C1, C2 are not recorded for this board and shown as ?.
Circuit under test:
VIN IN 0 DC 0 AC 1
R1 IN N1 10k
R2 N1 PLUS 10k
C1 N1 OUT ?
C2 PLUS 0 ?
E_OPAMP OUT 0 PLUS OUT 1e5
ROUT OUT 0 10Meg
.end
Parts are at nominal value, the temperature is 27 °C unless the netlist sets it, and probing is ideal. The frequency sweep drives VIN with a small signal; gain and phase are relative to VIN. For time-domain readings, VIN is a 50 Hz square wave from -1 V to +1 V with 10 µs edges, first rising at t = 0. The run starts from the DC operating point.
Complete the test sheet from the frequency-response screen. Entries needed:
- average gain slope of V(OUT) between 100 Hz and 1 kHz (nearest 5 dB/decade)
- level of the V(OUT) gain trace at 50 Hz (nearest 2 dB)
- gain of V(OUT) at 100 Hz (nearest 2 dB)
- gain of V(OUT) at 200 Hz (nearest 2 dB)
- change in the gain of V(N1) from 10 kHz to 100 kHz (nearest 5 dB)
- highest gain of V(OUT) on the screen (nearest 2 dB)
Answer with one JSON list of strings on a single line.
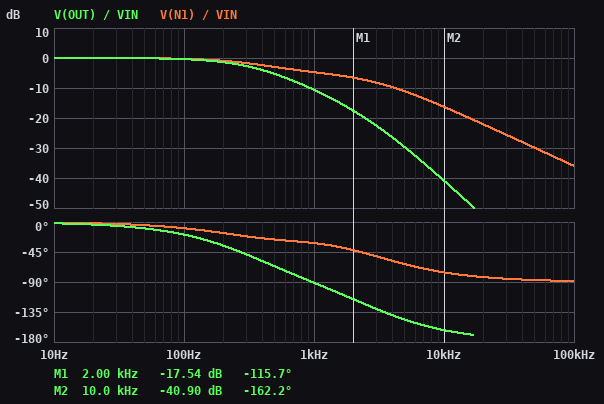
["-10 dB/decade", "0 dB", "0 dB", "-2 dB", "-20 dB", "0 dB"]
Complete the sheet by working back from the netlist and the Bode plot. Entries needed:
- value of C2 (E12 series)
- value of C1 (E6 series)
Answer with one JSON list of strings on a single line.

["27 nF", "10 nF"]
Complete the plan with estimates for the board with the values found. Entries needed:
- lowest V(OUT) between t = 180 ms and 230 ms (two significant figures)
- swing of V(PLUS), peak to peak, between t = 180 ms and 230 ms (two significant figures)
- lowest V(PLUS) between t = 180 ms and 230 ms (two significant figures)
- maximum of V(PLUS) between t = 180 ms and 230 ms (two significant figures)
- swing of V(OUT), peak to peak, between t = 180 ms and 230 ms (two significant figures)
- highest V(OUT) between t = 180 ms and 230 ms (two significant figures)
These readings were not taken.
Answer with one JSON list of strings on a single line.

["-1.0 V", "2.0 V", "-1.0 V", "1.0 V", "2.0 V", "1.0 V"]
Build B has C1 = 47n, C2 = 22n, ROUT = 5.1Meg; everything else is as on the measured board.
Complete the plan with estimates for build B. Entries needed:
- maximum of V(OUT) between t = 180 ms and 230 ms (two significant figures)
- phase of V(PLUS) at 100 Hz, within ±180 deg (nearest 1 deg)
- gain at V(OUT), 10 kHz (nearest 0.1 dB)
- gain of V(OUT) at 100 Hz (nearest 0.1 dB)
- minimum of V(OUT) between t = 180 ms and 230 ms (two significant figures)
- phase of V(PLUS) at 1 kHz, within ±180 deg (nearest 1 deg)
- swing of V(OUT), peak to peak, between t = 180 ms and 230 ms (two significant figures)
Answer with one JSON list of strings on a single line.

["1.1 V", "-16 deg", "-52.2 dB", "0 dB", "-1.1 V", "-138 deg", "2.2 V"]
